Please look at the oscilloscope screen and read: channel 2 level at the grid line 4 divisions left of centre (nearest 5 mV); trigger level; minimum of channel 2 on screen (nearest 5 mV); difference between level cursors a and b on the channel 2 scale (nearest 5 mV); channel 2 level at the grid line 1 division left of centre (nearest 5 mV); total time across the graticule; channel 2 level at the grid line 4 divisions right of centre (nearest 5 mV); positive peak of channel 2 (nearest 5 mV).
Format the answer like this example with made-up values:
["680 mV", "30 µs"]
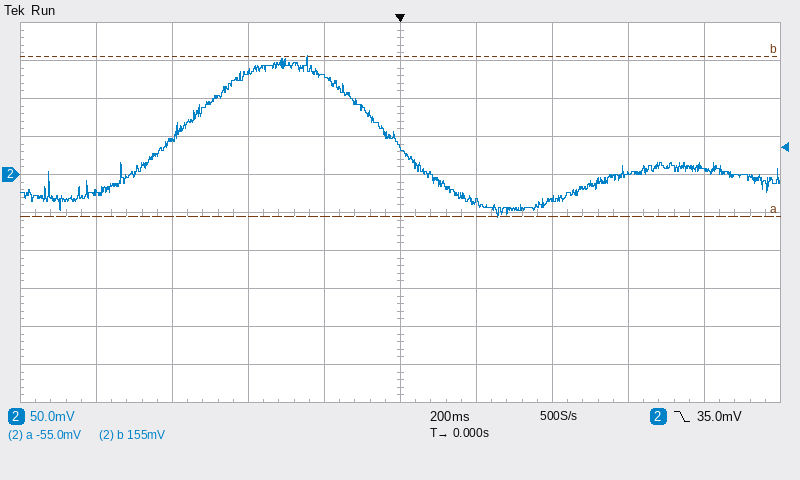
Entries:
["-25 mV", "35.0 mV", "-55 mV", "210 mV", "130 mV", "2 s", "10 mV", "155 mV"]
